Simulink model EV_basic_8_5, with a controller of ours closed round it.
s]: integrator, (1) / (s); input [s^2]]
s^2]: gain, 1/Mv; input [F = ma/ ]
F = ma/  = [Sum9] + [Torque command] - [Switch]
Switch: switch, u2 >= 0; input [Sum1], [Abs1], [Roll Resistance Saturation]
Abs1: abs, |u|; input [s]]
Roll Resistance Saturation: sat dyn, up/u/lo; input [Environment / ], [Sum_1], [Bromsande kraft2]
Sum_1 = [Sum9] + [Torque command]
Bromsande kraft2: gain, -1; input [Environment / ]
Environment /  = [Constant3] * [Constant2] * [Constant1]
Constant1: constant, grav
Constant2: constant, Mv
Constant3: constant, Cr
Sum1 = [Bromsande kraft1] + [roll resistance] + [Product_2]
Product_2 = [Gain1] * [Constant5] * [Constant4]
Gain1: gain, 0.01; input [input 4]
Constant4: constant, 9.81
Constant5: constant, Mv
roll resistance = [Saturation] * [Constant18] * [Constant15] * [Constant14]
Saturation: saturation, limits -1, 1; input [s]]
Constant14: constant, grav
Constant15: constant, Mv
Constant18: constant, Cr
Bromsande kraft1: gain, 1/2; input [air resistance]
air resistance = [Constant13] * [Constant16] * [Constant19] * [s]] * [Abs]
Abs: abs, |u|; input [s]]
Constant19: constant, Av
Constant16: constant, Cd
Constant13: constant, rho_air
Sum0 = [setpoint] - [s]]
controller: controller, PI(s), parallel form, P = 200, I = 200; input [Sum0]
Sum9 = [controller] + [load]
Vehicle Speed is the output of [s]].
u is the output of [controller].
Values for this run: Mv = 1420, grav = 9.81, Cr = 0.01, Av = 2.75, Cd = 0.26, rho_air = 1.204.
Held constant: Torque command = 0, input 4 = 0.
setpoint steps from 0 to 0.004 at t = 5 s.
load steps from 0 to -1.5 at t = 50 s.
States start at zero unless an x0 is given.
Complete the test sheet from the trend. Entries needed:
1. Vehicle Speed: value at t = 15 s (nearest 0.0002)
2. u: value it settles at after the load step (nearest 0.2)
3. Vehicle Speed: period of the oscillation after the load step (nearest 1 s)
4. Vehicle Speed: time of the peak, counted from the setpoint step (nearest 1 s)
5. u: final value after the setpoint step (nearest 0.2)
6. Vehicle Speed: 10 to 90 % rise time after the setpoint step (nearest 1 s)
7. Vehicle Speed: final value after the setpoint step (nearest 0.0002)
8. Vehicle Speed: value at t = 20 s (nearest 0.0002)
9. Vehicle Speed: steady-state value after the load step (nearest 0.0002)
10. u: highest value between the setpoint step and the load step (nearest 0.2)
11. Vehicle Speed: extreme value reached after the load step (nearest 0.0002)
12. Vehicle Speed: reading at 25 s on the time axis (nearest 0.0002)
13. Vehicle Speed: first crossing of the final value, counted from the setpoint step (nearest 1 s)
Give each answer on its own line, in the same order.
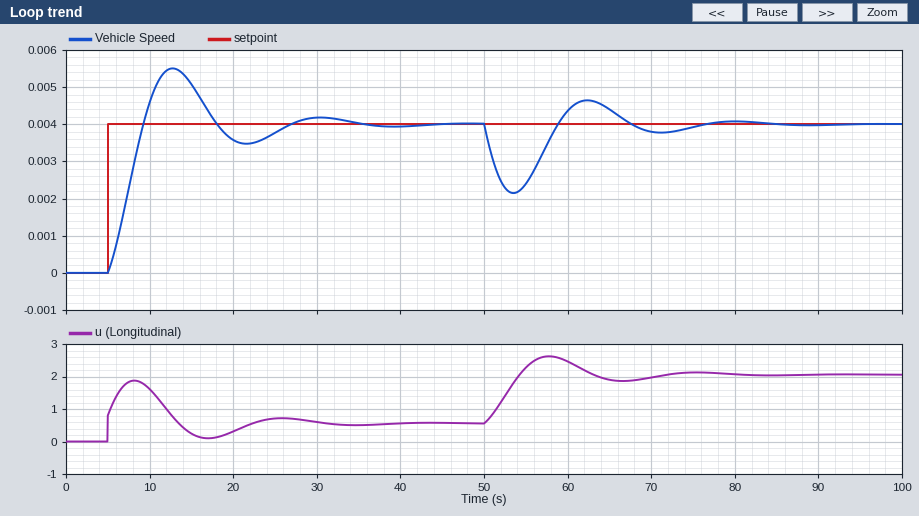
0.0050
2.0
18 s
8 s
0.6
3 s
0.0040
0.0036
0.0040
1.8
0.0022
0.0038
4 s
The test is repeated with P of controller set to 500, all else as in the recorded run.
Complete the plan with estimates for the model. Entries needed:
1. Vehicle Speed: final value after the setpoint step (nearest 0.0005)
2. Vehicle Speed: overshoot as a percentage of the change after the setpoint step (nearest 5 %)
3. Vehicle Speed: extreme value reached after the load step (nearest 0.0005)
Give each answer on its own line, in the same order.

0.0040
20 %
0.0025
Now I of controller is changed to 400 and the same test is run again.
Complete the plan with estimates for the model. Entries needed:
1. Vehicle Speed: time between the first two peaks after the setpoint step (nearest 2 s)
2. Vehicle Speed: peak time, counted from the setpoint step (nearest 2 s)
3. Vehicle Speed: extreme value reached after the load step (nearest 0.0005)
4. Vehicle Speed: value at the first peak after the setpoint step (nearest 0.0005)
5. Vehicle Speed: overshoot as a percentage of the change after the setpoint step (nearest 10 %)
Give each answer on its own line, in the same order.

12 s
6 s
0.0025
0.0060
50 %
